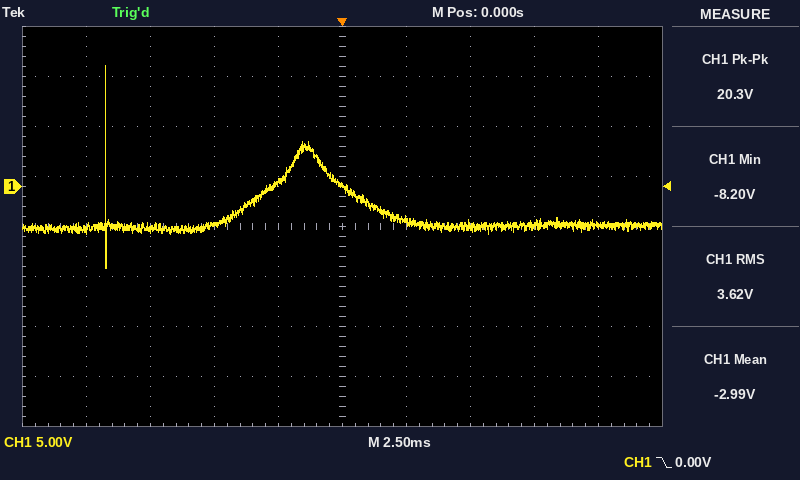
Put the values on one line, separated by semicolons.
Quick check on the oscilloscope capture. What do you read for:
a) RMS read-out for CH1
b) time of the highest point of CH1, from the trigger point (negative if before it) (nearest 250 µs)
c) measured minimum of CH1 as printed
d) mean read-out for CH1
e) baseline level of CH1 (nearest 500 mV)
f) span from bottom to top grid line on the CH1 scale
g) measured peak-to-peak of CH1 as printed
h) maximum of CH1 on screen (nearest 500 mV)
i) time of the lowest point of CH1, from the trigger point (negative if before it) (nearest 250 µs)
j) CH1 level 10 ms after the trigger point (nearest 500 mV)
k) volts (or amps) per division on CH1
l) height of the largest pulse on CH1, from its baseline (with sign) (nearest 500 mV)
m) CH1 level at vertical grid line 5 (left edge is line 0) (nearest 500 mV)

3.62 V; -9.25 ms; -8.20 V; -2.99 V; -4.0 V; 40 V; 20.3 V; 12.0 V; -9.25 ms; -4.0 V; 5 V; +16.0 V; 0.0 V
